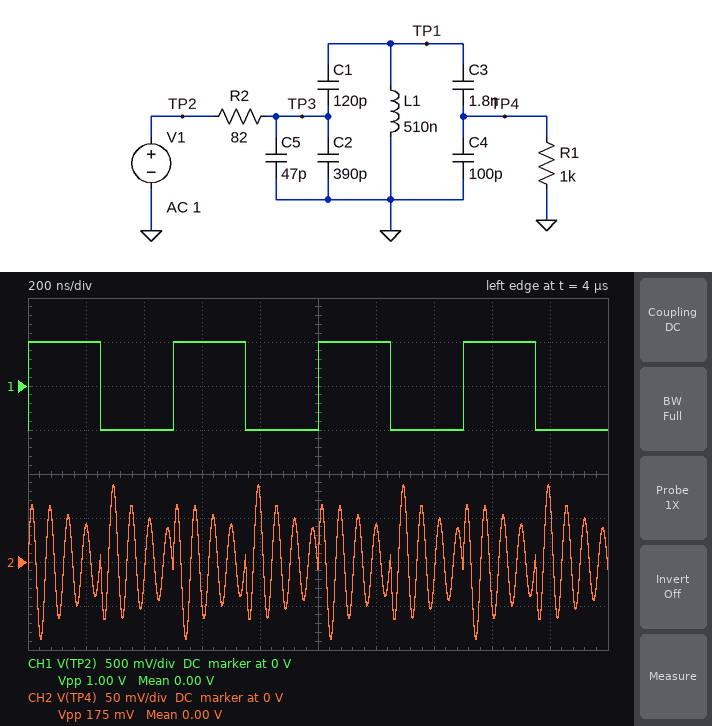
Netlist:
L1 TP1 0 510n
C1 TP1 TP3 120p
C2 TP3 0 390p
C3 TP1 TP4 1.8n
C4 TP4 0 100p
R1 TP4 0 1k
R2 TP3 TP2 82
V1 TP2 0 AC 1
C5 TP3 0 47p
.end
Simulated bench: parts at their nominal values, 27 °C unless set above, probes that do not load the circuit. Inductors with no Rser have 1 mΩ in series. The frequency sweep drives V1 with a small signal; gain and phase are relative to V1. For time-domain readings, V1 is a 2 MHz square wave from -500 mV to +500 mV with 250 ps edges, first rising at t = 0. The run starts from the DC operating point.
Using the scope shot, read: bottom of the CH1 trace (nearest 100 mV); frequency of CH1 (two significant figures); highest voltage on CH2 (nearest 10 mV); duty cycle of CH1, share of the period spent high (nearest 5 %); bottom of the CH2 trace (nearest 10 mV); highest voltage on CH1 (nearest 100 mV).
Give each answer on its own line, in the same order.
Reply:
-500 mV
2.0 MHz
90 mV
50 %
-90 mV
500 mV
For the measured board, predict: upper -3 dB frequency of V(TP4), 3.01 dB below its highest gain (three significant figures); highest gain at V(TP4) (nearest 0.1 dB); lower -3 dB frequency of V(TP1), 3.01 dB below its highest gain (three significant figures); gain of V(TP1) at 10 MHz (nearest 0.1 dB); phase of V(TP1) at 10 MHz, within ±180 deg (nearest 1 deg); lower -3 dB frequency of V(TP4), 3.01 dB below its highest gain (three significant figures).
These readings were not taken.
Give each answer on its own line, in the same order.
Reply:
16.8 MHz
4.6 dB
15.6 MHz
-17.8 dB
105 deg
15.6 MHz
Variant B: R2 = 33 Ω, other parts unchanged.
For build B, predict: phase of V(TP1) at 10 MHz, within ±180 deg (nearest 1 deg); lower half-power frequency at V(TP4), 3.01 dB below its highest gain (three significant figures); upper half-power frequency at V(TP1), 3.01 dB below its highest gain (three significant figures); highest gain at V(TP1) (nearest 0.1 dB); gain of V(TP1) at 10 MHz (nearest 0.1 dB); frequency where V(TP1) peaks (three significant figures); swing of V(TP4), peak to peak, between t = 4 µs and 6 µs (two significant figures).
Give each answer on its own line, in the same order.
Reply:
126 deg
15.2 MHz
16.8 MHz
9.2 dB
-11.6 dB
16.0 MHz
400 mV
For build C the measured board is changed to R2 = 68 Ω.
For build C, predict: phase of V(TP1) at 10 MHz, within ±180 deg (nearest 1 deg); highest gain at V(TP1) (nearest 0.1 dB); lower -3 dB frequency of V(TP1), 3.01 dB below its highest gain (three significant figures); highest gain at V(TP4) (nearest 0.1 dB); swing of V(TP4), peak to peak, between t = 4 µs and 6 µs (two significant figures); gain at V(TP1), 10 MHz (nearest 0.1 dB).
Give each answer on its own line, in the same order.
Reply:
108 deg
6.0 dB
15.5 MHz
5.5 dB
210 mV
-16.3 dB
